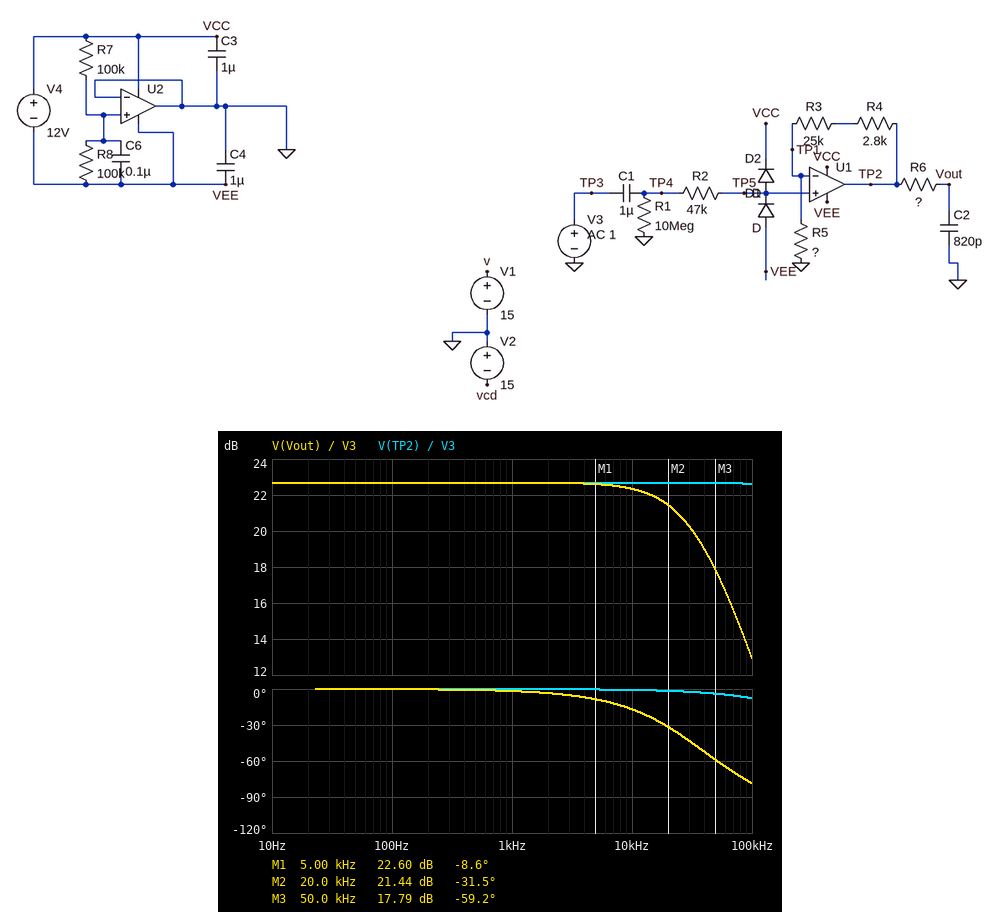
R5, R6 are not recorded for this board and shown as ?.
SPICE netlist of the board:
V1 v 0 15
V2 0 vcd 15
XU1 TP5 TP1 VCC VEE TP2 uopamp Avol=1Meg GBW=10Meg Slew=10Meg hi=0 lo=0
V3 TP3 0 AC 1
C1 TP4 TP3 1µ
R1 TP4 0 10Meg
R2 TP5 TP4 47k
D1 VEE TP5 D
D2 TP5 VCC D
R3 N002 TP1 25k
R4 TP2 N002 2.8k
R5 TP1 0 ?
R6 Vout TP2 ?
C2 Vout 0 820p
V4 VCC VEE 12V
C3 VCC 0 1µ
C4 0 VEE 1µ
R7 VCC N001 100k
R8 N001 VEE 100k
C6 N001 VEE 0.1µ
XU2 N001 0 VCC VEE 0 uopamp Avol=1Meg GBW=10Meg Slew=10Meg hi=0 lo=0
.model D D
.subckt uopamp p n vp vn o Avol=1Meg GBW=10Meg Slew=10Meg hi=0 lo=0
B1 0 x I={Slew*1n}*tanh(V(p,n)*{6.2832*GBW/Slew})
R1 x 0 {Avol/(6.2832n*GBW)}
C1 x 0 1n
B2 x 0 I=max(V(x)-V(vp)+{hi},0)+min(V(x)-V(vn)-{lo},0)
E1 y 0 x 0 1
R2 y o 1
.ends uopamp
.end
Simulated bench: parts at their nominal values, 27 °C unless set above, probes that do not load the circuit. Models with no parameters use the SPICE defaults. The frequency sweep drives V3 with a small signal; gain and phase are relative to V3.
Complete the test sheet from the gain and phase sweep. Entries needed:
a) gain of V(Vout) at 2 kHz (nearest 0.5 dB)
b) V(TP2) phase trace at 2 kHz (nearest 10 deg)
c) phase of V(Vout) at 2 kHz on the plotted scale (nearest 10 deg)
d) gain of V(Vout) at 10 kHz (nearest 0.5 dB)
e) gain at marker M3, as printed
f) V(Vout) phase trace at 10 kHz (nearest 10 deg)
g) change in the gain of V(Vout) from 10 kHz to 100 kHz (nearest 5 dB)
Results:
22.5 dB
0 deg
0 deg
22.5 dB
17.79 dB
-20 deg
-10 dB
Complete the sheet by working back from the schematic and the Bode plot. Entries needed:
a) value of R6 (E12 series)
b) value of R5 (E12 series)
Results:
5.6 kΩ
2.2 kΩ
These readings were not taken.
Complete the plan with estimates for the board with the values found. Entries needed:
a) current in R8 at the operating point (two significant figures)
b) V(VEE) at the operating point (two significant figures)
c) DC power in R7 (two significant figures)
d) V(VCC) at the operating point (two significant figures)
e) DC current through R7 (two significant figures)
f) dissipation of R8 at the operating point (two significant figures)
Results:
60 µA
-6.0 V
360 µW
6.0 V
60 µA
360 µW
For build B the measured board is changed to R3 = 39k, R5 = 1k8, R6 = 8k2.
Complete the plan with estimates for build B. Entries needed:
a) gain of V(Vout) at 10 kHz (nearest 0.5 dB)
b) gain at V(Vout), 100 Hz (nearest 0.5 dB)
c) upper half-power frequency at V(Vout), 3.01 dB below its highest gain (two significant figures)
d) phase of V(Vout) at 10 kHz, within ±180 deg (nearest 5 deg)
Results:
27.0 dB
27.5 dB
24 kHz
-25 deg
